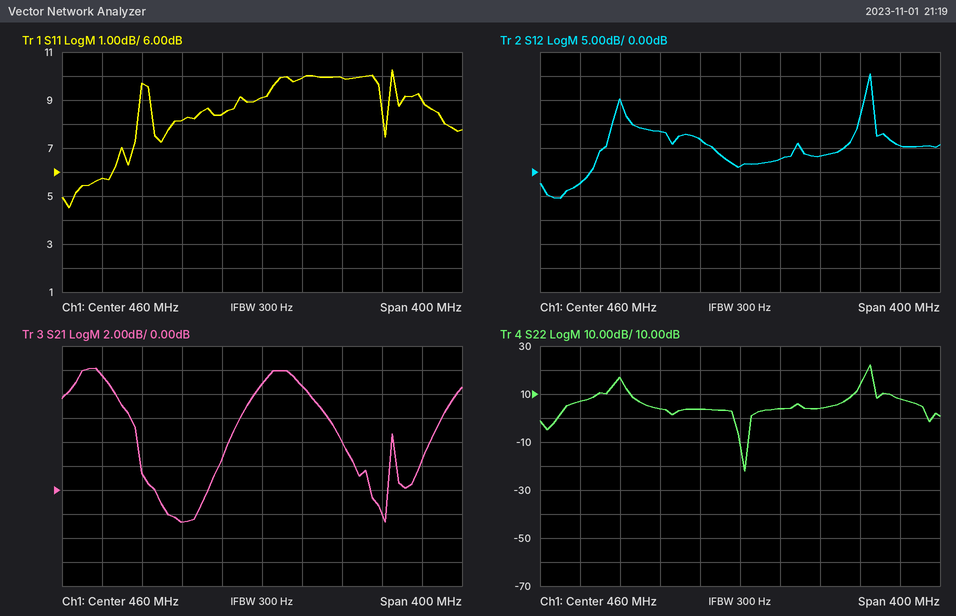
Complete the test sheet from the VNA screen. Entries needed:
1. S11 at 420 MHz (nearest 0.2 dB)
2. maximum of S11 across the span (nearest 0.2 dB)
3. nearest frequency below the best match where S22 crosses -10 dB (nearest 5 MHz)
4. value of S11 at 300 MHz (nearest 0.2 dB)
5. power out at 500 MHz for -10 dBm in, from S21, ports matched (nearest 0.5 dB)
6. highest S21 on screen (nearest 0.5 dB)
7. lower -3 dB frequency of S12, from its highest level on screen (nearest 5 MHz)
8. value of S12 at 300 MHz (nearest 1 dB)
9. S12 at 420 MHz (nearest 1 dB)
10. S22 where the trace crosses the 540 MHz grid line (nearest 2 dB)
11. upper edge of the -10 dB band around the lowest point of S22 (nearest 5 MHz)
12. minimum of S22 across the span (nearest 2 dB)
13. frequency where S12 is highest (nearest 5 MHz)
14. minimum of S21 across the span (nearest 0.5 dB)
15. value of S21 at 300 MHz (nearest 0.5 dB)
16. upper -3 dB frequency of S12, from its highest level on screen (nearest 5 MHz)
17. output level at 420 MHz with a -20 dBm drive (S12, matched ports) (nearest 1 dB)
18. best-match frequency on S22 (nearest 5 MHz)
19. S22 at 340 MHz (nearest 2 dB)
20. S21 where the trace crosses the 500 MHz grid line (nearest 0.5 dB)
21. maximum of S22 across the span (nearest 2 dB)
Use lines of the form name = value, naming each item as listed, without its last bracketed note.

S11 at 420 MHz = 8.4 dB
maximum of S11 across the span = 10.2 dB
nearest frequency below the best match where S22 crosses -10 dB = 460 MHz
value of S11 at 300 MHz = 5.8 dB
power out at 500 MHz for -10 dBm in, from S21, ports matched = -1.5 dBm
highest S21 on screen = 10.0 dB
lower -3 dB frequency of S12, from its highest level on screen = 585 MHz
value of S12 at 300 MHz = -2 dB
S12 at 420 MHz = 7 dB
S22 where the trace crosses the 540 MHz grid line = 4 dB
upper edge of the -10 dB band around the lowest point of S22 = 470 MHz
minimum of S22 across the span = -22 dB
frequency where S12 is highest = 590 MHz
minimum of S21 across the span = -2.5 dB
value of S21 at 300 MHz = 9.5 dB
upper -3 dB frequency of S12, from its highest level on screen = 590 MHz
output level at 420 MHz with a -20 dBm drive (S12, matched ports) = -13 dBm
best-match frequency on S22 = 465 MHz
S22 at 340 MHz = 16 dB
S21 where the trace crosses the 500 MHz grid line = 8.5 dB
maximum of S22 across the span = 22 dB
